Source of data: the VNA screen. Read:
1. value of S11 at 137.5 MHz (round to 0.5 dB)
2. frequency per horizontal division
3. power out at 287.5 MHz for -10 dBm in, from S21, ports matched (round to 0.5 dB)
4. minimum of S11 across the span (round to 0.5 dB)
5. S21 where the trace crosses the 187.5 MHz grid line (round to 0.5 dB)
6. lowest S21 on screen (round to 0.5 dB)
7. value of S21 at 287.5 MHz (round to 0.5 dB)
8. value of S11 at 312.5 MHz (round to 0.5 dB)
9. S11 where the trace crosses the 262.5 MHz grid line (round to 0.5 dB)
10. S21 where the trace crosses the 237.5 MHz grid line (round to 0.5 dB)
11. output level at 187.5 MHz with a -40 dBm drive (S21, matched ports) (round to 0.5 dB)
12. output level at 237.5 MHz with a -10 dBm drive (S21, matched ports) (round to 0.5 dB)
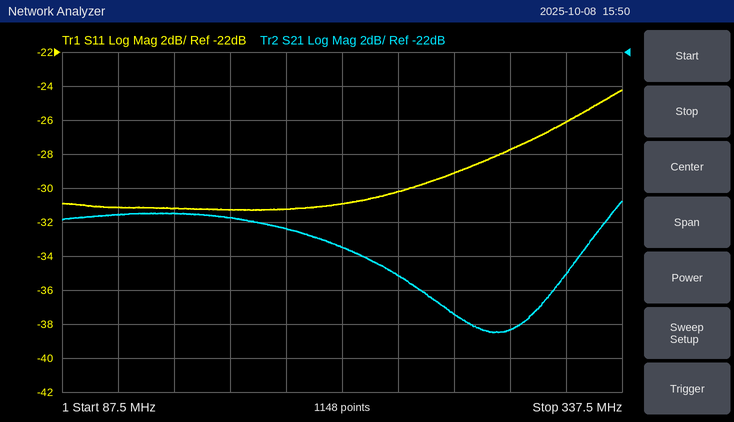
-31.0 dB
25 MHz
-48.5 dBm
-31.5 dB
-32.5 dB
-38.5 dB
-38.5 dB
-26.0 dB
-29.0 dB
-35.0 dB
-72.5 dBm
-45.0 dBm
